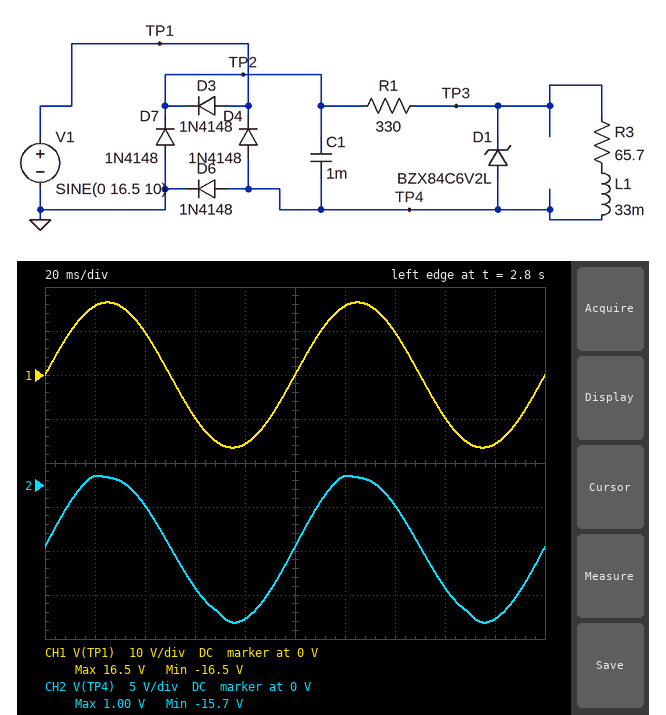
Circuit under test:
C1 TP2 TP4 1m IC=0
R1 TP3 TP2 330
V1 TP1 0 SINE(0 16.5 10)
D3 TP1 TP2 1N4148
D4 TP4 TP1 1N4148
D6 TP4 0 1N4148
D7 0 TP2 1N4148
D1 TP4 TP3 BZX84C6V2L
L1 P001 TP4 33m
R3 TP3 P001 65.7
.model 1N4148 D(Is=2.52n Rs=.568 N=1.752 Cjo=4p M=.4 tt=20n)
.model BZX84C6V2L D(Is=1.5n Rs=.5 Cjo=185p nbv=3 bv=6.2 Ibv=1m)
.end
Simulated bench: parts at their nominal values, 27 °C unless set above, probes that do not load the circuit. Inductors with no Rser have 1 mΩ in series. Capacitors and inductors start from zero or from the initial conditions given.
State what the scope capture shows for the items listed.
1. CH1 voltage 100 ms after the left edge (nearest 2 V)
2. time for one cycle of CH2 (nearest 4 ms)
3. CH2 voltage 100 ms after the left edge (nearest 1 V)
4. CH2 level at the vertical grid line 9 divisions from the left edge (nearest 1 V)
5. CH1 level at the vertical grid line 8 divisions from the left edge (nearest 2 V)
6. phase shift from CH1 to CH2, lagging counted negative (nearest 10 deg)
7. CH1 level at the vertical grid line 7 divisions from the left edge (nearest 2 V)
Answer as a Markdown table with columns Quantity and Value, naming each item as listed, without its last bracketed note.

| Quantity | Value |
|---|---|
| CH1 voltage 100 ms after the left edge | 0 V |
| time for one cycle of CH2 | 100 ms |
| CH2 voltage 100 ms after the left edge | -7 V |
| CH2 level at the vertical grid line 9 divisions from the left edge | -15 V |
| CH1 level at the vertical grid line 8 divisions from the left edge | -10 V |
| phase shift from CH1 to CH2, lagging counted negative | 0 deg |
| CH1 level at the vertical grid line 7 divisions from the left edge | 10 V |
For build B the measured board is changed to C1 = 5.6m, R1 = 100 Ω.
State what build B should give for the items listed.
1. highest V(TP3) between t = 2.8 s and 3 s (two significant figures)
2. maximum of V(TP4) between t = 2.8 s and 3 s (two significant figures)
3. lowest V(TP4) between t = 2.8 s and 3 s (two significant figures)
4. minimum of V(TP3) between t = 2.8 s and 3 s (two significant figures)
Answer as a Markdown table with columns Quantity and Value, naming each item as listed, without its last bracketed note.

| Quantity | Value |
|---|---|
| highest V(TP3) between t = 2.8 s and 3 s | 6.8 V |
| maximum of V(TP4) between t = 2.8 s and 3 s | 1.2 V |
| lowest V(TP4) between t = 2.8 s and 3 s | -15 V |
| minimum of V(TP3) between t = 2.8 s and 3 s | -9.7 V |
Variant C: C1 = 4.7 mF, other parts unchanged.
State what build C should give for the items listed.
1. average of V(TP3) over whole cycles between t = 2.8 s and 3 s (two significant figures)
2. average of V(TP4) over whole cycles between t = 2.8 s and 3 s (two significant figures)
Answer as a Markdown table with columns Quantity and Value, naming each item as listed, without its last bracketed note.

| Quantity | Value |
|---|---|
| average of V(TP3) over whole cycles between t = 2.8 s and 3 s | -4.8 V |
| average of V(TP4) over whole cycles between t = 2.8 s and 3 s | -7.2 V |
